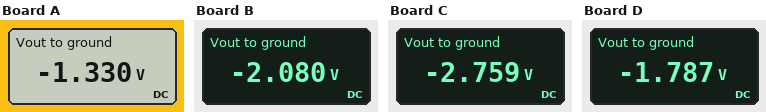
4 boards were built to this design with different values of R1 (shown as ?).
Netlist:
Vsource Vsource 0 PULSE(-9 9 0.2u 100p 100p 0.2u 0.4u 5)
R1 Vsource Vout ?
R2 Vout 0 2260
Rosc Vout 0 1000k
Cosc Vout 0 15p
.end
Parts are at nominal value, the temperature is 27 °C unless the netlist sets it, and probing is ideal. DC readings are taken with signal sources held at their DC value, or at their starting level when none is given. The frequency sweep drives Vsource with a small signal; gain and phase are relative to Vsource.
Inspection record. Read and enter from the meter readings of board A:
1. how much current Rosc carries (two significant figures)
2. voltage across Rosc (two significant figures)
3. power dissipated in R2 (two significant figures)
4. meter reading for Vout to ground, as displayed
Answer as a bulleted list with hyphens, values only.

- 1.3 µA
- 1.3 V
- 780 µW
- -1.330 V
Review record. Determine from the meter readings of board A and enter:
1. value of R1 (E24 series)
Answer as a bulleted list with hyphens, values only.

- 13 kΩ
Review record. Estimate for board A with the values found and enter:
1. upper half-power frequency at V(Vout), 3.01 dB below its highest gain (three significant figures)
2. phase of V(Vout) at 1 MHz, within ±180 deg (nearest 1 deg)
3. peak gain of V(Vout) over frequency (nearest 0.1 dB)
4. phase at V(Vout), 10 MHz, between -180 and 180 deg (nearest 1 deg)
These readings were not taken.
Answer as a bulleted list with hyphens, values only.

- 5.52 MHz
- -10 deg
- -16.6 dB
- -61 deg
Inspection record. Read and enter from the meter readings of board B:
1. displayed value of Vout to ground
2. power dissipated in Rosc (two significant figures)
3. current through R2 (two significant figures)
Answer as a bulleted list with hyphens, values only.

- -2.080 V
- 4.3 µW
- 920 µA
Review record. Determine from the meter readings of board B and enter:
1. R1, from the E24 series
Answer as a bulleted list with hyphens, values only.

- 7.5 kΩ
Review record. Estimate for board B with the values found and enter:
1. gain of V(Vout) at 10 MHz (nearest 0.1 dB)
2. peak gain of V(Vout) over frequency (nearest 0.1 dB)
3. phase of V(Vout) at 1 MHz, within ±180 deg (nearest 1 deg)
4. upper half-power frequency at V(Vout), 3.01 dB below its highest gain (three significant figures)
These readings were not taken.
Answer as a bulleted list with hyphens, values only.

- -18.4 dB
- -12.7 dB
- -9 deg
- 6.12 MHz
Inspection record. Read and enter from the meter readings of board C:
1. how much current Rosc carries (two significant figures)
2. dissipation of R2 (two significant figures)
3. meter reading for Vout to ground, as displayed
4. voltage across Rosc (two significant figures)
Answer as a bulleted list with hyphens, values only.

- 2.8 µA
- 3.4 mW
- -2.759 V
- 2.8 V
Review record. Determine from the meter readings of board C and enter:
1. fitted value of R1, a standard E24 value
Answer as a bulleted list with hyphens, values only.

- 5.1 kΩ
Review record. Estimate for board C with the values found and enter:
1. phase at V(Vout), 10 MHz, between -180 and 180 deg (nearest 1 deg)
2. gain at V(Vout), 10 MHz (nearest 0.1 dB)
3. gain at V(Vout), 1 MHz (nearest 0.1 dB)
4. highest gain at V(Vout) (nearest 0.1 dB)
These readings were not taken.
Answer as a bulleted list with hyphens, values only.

- -56 deg
- -15.3 dB
- -10.4 dB
- -10.3 dB
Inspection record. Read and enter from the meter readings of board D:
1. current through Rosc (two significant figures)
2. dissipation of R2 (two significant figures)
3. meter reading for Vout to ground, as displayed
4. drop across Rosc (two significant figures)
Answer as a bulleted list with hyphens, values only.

- 1.8 µA
- 1.4 mW
- -1.787 V
- 1.8 V
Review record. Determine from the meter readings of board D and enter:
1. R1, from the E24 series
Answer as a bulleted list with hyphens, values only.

- 9.1 kΩ
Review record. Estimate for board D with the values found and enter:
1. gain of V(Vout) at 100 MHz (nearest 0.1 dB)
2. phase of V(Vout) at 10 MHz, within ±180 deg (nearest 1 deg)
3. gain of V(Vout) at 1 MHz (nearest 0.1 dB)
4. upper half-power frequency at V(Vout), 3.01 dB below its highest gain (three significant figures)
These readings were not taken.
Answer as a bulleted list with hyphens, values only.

- -38.7 dB
- -60 deg
- -14.2 dB
- 5.87 MHz
